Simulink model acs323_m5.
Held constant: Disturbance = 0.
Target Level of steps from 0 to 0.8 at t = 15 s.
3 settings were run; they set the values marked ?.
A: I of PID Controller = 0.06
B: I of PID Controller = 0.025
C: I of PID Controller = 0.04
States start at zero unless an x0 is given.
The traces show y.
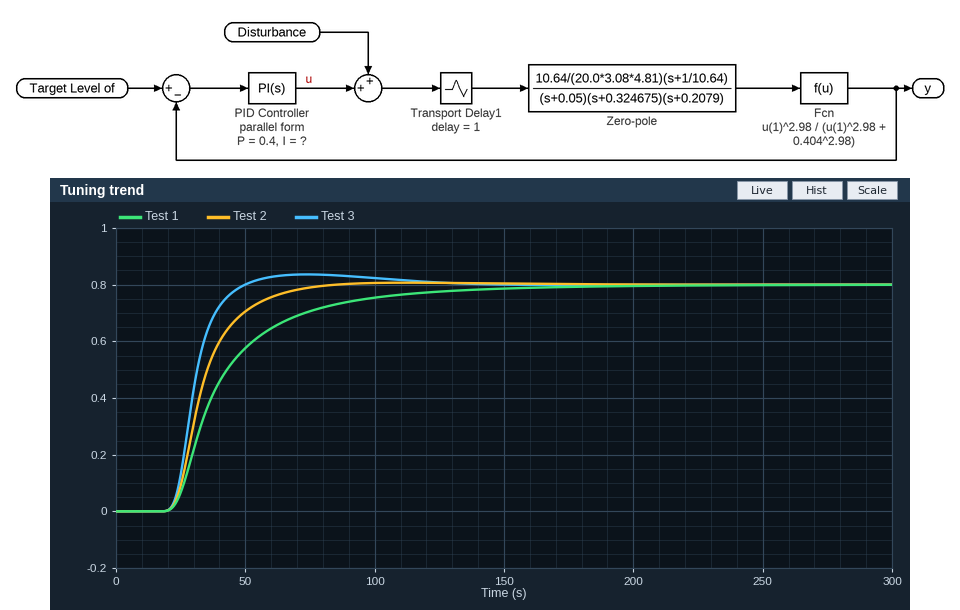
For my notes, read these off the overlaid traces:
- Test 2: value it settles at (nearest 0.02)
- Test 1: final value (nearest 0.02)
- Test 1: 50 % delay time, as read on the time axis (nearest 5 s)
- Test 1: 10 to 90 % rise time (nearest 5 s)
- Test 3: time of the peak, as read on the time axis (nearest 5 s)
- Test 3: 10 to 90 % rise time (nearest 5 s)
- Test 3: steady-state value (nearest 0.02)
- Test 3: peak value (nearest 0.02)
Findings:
0.80
0.80
35 s
55 s
75 s
15 s
0.80
0.84
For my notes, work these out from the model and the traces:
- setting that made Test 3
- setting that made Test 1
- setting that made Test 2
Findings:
A
B
C
